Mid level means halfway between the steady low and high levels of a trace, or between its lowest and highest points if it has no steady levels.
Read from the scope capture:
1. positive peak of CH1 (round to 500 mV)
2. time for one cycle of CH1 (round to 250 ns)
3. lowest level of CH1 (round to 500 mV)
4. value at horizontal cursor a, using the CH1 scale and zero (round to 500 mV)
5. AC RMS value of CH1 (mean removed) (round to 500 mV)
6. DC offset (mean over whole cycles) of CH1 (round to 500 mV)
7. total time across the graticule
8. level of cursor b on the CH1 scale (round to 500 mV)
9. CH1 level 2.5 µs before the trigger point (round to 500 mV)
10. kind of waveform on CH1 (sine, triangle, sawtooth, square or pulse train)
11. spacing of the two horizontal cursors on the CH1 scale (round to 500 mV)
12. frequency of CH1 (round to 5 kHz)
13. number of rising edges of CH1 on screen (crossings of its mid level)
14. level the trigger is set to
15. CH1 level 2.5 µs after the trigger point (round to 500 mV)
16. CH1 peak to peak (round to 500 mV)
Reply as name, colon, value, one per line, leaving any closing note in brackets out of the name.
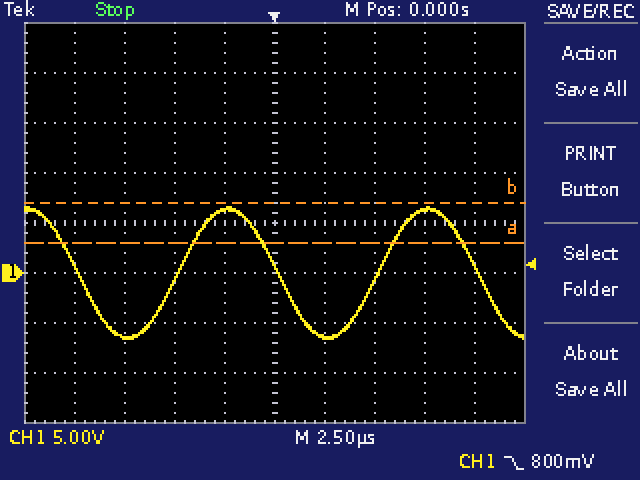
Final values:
positive peak of CH1: 6.5 V
time for one cycle of CH1: 10.00 µs
lowest level of CH1: -6.5 V
value at horizontal cursor a, using the CH1 scale and zero: 3.0 V
AC RMS value of CH1 (mean removed): 4.5 V
DC offset (mean over whole cycles) of CH1: 0.0 V
total time across the graticule: 25 µs
level of cursor b on the CH1 scale: 7.0 V
CH1 level 2.5 µs before the trigger point: 6.5 V
kind of waveform on CH1: sine
spacing of the two horizontal cursors on the CH1 scale: 4.0 V
frequency of CH1: 100 kHz
number of rising edges of CH1 on screen: 2
level the trigger is set to: 800 mV
CH1 level 2.5 µs after the trigger point: -6.5 V
CH1 peak to peak: 13.0 V
